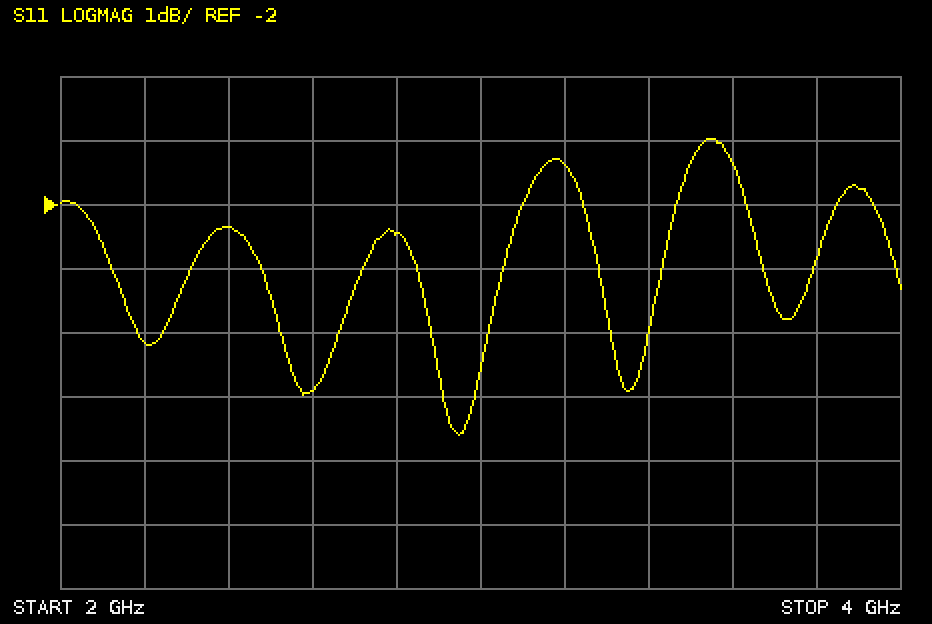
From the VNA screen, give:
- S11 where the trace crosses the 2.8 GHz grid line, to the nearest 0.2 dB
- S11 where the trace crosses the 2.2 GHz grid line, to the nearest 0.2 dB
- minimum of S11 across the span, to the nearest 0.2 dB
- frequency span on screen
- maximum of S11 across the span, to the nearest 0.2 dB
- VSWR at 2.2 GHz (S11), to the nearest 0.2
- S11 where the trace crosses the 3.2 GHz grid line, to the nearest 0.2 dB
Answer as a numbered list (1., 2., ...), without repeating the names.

1. -2.4 dB
2. -4.2 dB
3. -5.6 dB
4. 2 GHz
5. -1.0 dB
6. 4.2
7. -1.4 dB
